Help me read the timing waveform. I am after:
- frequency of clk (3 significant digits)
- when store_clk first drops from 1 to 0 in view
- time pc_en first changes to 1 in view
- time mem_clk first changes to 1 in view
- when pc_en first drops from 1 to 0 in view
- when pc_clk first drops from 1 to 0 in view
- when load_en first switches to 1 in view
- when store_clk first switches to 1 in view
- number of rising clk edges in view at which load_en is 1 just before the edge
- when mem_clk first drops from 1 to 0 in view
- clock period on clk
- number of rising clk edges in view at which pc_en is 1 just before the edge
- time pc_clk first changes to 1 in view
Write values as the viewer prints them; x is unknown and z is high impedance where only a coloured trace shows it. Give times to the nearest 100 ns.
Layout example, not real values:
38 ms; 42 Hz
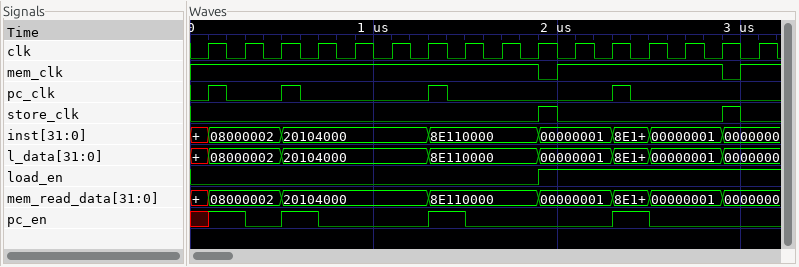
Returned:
5.00 MHz; 2000 ns; 100 ns; 2000 ns; 300 ns; 200 ns; 1900 ns; 1900 ns; 6; 1900 ns; 200 ns; 4; 100 ns
